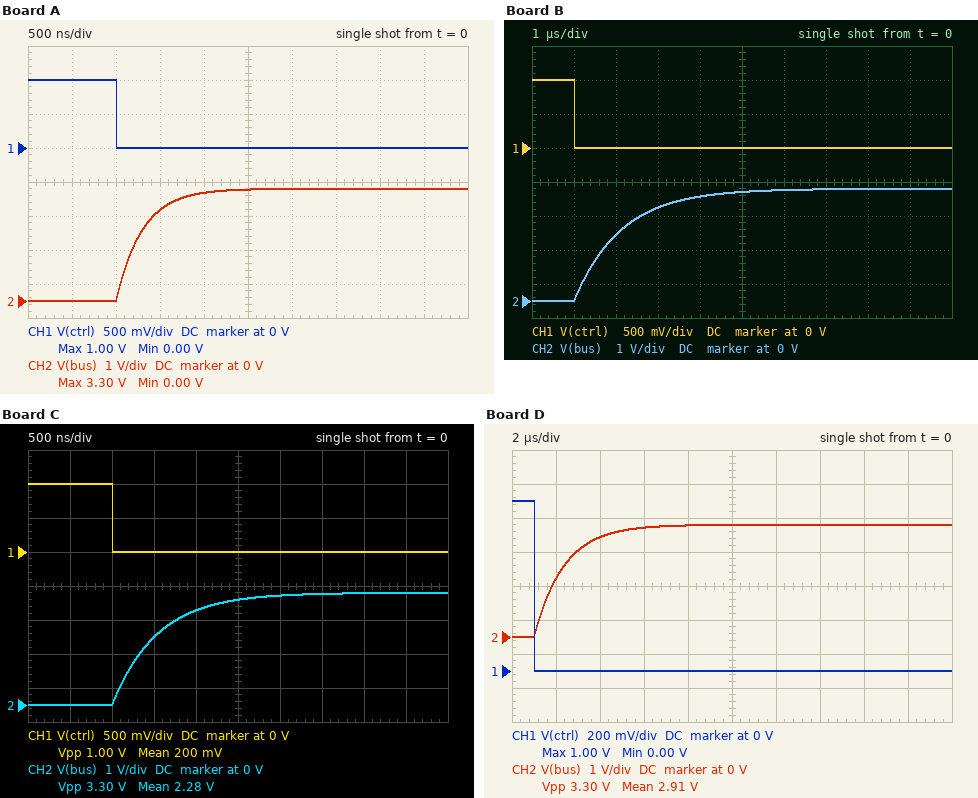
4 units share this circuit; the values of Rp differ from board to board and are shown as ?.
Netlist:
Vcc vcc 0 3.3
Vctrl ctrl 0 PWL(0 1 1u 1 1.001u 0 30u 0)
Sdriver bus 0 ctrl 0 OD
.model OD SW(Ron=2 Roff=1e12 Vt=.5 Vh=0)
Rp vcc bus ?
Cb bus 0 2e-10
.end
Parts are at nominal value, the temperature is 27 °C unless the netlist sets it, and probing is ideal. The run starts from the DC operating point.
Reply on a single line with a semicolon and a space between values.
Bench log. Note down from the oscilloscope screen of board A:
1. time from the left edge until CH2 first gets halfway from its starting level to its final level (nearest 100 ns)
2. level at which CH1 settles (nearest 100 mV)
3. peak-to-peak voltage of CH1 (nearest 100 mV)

1.2 µs; 0 V; 1.0 V
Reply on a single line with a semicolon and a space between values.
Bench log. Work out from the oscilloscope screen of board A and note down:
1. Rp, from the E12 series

1.5 kΩ
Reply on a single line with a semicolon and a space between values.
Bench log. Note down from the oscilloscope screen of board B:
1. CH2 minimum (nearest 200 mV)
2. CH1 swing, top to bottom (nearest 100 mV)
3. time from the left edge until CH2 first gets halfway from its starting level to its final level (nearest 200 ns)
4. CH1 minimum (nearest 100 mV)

0 V; 1.0 V; 1.8 µs; 0 V
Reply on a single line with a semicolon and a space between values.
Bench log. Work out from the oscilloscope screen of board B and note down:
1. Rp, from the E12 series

5.6 kΩ
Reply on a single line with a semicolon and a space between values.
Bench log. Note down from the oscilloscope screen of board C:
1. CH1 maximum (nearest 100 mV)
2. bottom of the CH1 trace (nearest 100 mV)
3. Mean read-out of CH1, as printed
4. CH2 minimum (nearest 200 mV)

1.0 V; 0 V; 200 mV; 0 V
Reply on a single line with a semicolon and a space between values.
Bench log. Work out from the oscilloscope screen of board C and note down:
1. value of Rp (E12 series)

2.7 kΩ
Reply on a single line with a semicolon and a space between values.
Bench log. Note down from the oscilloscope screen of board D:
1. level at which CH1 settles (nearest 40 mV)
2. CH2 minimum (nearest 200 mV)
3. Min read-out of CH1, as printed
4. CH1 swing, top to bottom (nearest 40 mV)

0 V; 0 V; 0.00 V; 1.00 V
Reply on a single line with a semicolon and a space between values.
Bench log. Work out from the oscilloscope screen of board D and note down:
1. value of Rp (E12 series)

6.8 kΩ
